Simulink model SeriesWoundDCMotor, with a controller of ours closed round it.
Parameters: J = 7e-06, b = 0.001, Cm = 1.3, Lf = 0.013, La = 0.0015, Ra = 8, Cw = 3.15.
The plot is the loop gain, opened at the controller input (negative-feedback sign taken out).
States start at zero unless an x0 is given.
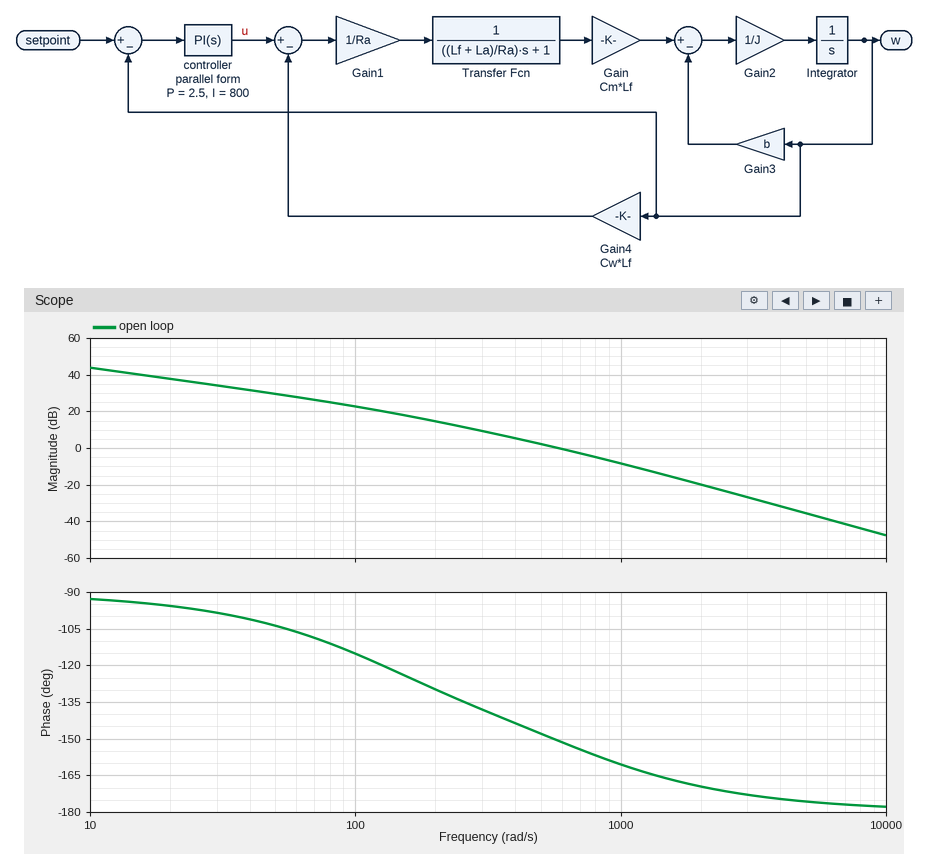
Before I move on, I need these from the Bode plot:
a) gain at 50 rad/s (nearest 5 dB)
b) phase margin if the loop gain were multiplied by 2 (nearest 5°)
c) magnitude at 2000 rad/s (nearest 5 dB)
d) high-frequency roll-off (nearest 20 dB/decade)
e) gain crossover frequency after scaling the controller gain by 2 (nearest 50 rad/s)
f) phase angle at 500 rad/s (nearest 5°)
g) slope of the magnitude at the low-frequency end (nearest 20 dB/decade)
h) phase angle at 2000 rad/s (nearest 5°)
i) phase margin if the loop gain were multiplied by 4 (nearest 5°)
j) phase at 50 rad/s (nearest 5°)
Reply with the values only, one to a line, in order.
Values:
30 dB
20°
-20 dB
-40 dB/decade
850 rad/s
-150°
-20 dB/decade
-170°
15°
-105°
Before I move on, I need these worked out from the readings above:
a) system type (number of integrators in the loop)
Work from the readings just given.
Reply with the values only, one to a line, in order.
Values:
1
